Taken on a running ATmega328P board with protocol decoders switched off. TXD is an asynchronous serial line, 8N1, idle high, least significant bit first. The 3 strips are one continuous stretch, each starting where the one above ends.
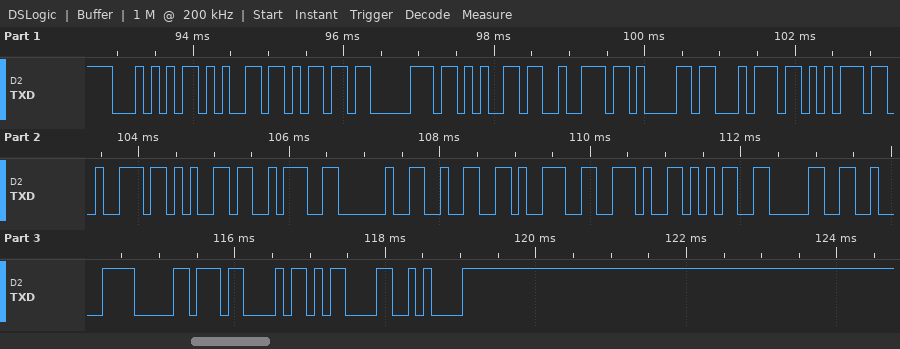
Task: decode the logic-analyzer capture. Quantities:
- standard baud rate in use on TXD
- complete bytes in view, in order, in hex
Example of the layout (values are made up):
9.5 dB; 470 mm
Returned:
9600 baud; 54 65 6D 70 65 72 61 74 75 72 65 3A 20 32 39 2E 35 30 C2 B0 43 0D 0A
